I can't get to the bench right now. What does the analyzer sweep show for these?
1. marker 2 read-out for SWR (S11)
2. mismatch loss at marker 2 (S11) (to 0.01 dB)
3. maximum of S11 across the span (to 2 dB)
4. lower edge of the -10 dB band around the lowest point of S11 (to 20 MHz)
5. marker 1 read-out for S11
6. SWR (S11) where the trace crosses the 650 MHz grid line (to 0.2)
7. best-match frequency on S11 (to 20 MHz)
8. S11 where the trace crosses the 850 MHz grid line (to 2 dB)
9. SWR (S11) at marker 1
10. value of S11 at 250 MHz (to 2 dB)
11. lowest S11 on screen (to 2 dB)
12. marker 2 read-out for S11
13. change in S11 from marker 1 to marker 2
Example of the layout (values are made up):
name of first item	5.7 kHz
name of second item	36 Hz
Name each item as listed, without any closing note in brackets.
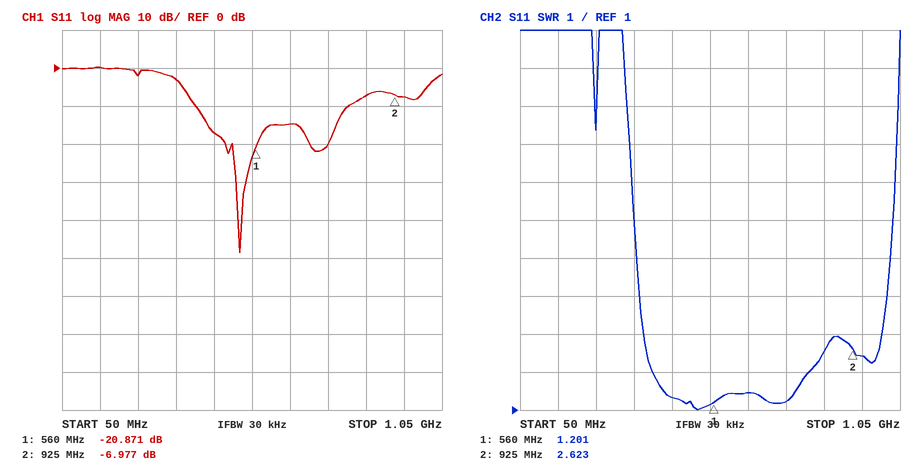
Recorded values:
marker 2 read-out for SWR	2.623
mismatch loss at marker 2 (S11)	0.97 dB
maximum of S11 across the span	0 dB
lower edge of the -10 dB band around the lowest point of S11	400 MHz
marker 1 read-out for S11	-20.871 dB
SWR (S11) where the trace crosses the 650 MHz grid line	1.4
best-match frequency on S11	520 MHz
S11 where the trace crosses the 850 MHz grid line	-8 dB
SWR (S11) at marker 1	1.201
value of S11 at 250 MHz	-2 dB
lowest S11 on screen	-48 dB
marker 2 read-out for S11	-6.977 dB
change in S11 from marker 1 to marker 2	13.894 dB
